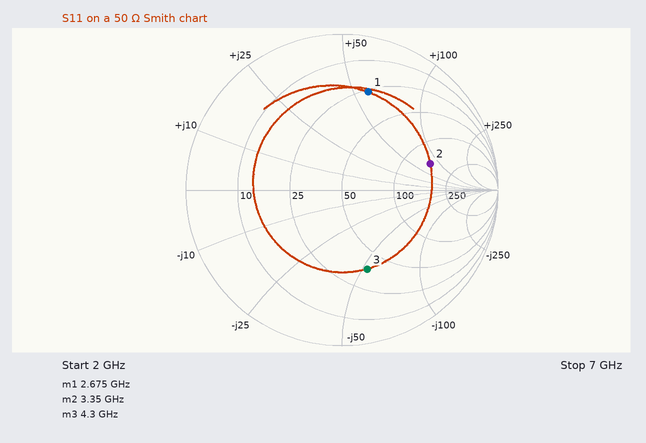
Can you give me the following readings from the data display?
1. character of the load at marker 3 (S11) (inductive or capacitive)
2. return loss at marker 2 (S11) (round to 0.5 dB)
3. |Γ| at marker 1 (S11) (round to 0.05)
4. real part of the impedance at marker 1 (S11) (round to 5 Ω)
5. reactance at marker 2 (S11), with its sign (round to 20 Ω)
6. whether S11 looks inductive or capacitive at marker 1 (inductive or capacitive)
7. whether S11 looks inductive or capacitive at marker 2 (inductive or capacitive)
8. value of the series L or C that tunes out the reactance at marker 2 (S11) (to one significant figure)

capacitive
4.5 dB
0.65
25 Ω
+80 Ω
inductive
inductive
600 fF
